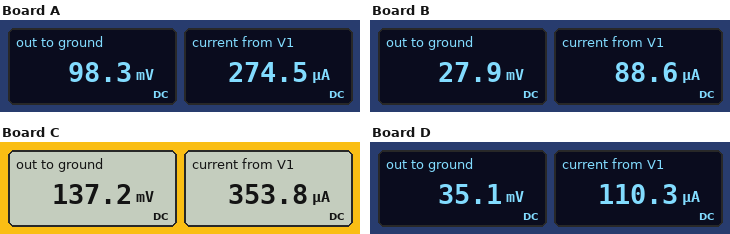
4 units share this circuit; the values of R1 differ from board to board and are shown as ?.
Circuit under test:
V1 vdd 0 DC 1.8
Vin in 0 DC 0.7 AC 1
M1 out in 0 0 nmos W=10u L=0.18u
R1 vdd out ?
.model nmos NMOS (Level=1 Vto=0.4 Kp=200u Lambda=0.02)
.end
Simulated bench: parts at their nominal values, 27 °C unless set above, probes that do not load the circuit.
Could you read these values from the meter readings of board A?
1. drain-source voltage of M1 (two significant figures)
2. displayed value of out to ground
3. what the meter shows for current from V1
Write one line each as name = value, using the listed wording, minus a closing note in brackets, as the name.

drain-source voltage of M1 = 98 mV
displayed value of out to ground = 98.3 mV
what the meter shows for current from V1 = 274.5 µA
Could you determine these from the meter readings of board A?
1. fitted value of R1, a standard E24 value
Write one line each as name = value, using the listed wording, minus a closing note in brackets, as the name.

fitted value of R1, a standard E24 value = 6.2 kΩ
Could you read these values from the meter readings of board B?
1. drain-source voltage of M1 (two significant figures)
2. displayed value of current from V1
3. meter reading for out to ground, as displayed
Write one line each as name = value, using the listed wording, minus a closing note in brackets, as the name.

drain-source voltage of M1 = 28 mV
displayed value of current from V1 = 88.6 µA
meter reading for out to ground, as displayed = 27.9 mV
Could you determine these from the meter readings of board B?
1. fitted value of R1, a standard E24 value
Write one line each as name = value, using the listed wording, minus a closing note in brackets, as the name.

fitted value of R1, a standard E24 value = 20 kΩ
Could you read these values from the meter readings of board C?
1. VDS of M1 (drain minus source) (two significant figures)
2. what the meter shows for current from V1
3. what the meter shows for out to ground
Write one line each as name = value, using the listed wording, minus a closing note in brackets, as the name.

VDS of M1 (drain minus source) = 140 mV
what the meter shows for current from V1 = 353.8 µA
what the meter shows for out to ground = 137.2 mV
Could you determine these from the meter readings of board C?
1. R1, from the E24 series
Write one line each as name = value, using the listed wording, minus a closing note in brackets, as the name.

R1, from the E24 series = 4.7 kΩ
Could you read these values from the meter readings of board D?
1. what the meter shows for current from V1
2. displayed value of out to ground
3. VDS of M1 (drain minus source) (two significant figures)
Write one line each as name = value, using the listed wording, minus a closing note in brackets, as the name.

what the meter shows for current from V1 = 110.3 µA
displayed value of out to ground = 35.1 mV
VDS of M1 (drain minus source) = 35 mV
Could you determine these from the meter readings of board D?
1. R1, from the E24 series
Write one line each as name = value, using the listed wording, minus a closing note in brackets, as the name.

R1, from the E24 series = 16 kΩ
